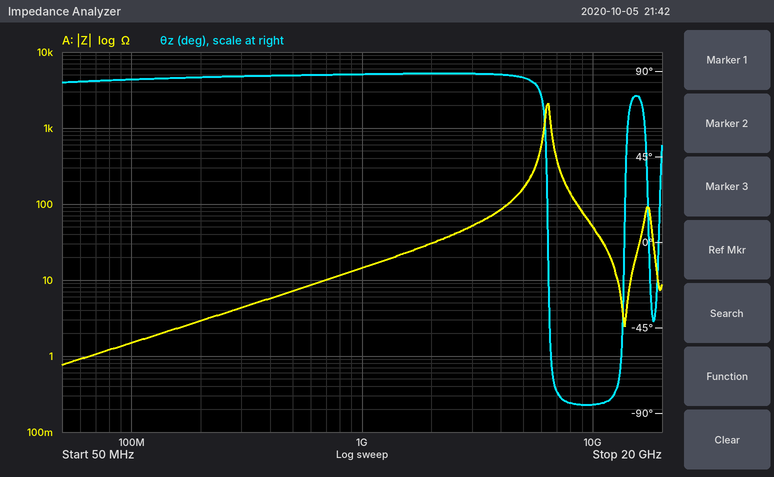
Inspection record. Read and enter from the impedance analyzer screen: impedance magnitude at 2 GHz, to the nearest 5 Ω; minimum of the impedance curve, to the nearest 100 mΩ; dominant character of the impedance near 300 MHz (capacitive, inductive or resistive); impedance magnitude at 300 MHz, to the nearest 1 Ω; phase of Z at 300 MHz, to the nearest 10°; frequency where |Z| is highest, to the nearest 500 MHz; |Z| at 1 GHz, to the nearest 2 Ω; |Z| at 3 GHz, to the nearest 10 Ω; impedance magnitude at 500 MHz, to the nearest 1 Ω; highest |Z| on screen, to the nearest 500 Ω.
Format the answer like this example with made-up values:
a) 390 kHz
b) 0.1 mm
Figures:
a) 30 Ω
b) 800 mΩ
c) inductive
d) 4 Ω
e) 90°
f) 6.5 GHz
g) 14 Ω
h) 50 Ω
i) 7 Ω
j) 2.0 kΩ
